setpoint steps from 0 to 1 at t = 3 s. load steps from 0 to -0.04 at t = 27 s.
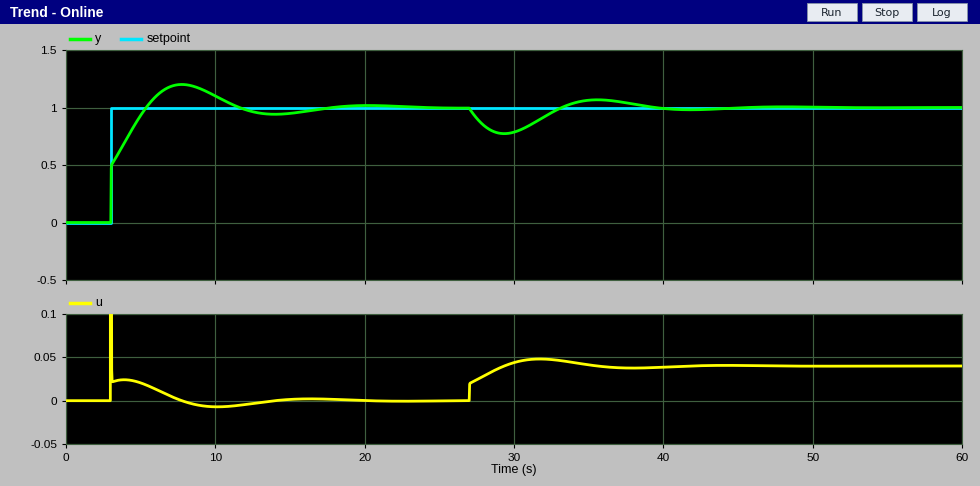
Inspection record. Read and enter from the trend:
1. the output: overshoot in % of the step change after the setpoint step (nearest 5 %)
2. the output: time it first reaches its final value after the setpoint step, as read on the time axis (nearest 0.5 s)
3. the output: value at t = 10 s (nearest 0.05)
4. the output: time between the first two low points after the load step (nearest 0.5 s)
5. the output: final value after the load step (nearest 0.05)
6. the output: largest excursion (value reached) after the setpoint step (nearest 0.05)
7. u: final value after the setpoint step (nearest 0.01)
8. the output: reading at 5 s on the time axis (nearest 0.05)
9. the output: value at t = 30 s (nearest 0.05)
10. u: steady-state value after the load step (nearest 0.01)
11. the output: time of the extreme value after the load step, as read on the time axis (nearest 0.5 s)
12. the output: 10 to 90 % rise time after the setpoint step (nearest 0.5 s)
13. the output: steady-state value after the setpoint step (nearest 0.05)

20 %
5.5 s
1.10
12.5 s
1.00
1.20
0.00
0.95
0.80
0.04
29.5 s
2.0 s
1.00
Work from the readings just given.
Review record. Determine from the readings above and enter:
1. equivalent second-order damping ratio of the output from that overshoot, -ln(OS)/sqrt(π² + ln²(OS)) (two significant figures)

0.46
